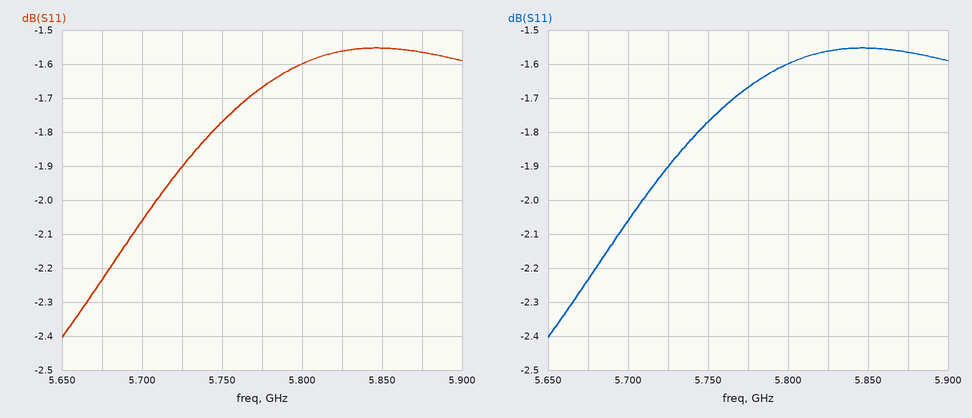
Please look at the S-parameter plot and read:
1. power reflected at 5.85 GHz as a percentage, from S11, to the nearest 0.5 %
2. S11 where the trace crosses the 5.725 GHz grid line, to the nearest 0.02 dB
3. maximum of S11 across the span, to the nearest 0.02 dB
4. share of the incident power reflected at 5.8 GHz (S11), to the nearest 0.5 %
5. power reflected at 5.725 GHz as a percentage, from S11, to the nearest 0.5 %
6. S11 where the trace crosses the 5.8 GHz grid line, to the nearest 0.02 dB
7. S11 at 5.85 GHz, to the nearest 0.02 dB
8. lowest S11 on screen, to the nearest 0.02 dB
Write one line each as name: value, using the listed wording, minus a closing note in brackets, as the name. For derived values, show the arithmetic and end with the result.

power reflected at 5.85 GHz as a percentage, from S11, to the nearest 0.5 %: 10^(-1.56/10) ≈ 69.8 %, so 70.0 % to the nearest 0.5 %
S11 where the trace crosses the 5.725 GHz grid line, to the nearest 0.02 dB: -1.90 dB
maximum of S11 across the span, to the nearest 0.02 dB: -1.56 dB
share of the incident power reflected at 5.8 GHz (S11), to the nearest 0.5 %: 10^(-1.6/10) ≈ 69.2 %, so 69.0 % to the nearest 0.5 %
power reflected at 5.725 GHz as a percentage, from S11, to the nearest 0.5 %: 10^(-1.9/10) ≈ 64.6 %, so 64.5 % to the nearest 0.5 %
S11 where the trace crosses the 5.8 GHz grid line, to the nearest 0.02 dB: -1.60 dB
S11 at 5.85 GHz, to the nearest 0.02 dB: -1.56 dB
lowest S11 on screen, to the nearest 0.02 dB: -2.40 dB
